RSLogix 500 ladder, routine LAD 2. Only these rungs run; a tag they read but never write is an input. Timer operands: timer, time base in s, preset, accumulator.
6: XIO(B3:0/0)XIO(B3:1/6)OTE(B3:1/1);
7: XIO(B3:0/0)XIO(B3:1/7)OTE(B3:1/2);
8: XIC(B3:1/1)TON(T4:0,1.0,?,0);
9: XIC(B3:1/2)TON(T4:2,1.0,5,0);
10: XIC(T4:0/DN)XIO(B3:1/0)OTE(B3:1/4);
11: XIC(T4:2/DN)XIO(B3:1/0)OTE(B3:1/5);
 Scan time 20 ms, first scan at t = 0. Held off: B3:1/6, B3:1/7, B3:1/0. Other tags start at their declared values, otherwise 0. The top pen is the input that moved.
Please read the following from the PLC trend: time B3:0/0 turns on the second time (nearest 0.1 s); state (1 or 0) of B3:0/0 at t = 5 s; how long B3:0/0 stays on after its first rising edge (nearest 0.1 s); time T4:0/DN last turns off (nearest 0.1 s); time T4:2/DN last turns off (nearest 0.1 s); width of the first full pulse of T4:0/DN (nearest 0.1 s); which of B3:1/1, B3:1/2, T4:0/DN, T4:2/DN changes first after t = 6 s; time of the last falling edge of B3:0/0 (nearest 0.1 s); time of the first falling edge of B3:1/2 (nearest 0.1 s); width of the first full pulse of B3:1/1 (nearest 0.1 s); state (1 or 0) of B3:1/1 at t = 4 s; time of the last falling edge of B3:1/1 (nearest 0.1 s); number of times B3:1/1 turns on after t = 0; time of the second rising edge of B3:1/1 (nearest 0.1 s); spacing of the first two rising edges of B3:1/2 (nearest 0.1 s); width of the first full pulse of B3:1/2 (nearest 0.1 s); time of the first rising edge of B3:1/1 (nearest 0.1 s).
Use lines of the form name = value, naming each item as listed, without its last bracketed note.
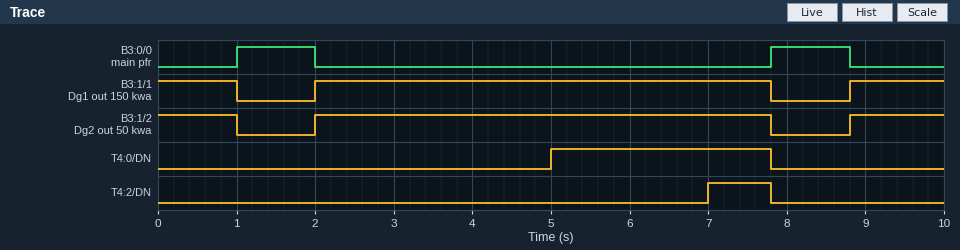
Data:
time B3:0/0 turns on the second time = 7.8 s
state (1 or 0) of B3:0/0 at t = 5 s = 0
how long B3:0/0 stays on after its first rising edge = 1.0 s
time T4:0/DN last turns off = 7.8 s
time T4:2/DN last turns off = 7.8 s
width of the first full pulse of T4:0/DN = 2.8 s
which of B3:1/1, B3:1/2, T4:0/DN, T4:2/DN changes first after t = 6 s = T4:2/DN
time of the last falling edge of B3:0/0 = 8.8 s
time of the first falling edge of B3:1/2 = 1.0 s
width of the first full pulse of B3:1/1 = 5.8 s
state (1 or 0) of B3:1/1 at t = 4 s = 1
time of the last falling edge of B3:1/1 = 7.8 s
number of times B3:1/1 turns on after t = 0 = 2
time of the second rising edge of B3:1/1 = 8.8 s
spacing of the first two rising edges of B3:1/2 = 6.8 s
width of the first full pulse of B3:1/2 = 5.8 s
time of the first rising edge of B3:1/1 = 2.0 s
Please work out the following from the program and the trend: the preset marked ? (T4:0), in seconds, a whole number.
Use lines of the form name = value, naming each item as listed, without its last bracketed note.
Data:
the preset marked ? (T4:0), in seconds, a whole number = 3 s
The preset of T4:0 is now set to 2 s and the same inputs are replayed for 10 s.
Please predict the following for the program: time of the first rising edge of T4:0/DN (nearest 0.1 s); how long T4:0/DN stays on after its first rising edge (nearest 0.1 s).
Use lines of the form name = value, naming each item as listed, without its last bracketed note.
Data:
time of the first rising edge of T4:0/DN = 4.0 s
how long T4:0/DN stays on after its first rising edge = 3.8 s
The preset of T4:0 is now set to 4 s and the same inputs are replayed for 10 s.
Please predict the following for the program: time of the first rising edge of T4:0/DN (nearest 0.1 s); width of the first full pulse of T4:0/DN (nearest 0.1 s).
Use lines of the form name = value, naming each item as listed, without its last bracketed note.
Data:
time of the first rising edge of T4:0/DN = 6.0 s
width of the first full pulse of T4:0/DN = 1.8 s
